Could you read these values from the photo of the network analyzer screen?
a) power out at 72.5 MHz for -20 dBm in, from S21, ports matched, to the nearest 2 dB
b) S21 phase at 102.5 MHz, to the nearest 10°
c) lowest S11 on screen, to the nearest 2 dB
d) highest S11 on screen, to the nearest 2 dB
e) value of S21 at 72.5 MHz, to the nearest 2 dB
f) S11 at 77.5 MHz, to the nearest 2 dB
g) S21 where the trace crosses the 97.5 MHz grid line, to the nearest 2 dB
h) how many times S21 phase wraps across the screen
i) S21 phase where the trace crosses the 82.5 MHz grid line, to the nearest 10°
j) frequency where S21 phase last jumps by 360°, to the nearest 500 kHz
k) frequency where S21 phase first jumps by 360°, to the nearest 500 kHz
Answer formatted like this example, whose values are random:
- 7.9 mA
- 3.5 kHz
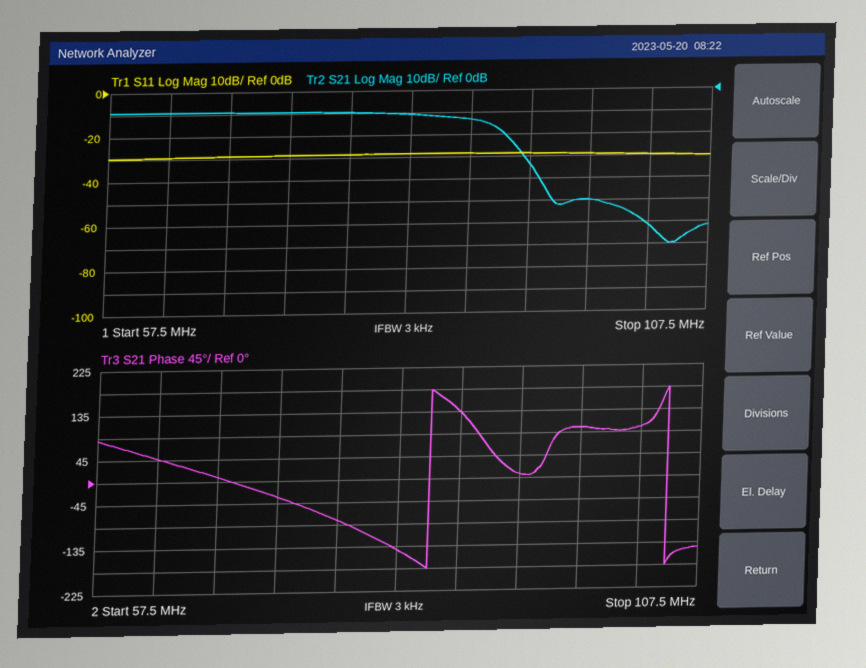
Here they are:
- -30 dBm
- 100°
- -30 dB
- -28 dB
- -10 dB
- -28 dB
- -50 dB
- 2
- -140°
- 105.0 MHz
- 85.0 MHz
